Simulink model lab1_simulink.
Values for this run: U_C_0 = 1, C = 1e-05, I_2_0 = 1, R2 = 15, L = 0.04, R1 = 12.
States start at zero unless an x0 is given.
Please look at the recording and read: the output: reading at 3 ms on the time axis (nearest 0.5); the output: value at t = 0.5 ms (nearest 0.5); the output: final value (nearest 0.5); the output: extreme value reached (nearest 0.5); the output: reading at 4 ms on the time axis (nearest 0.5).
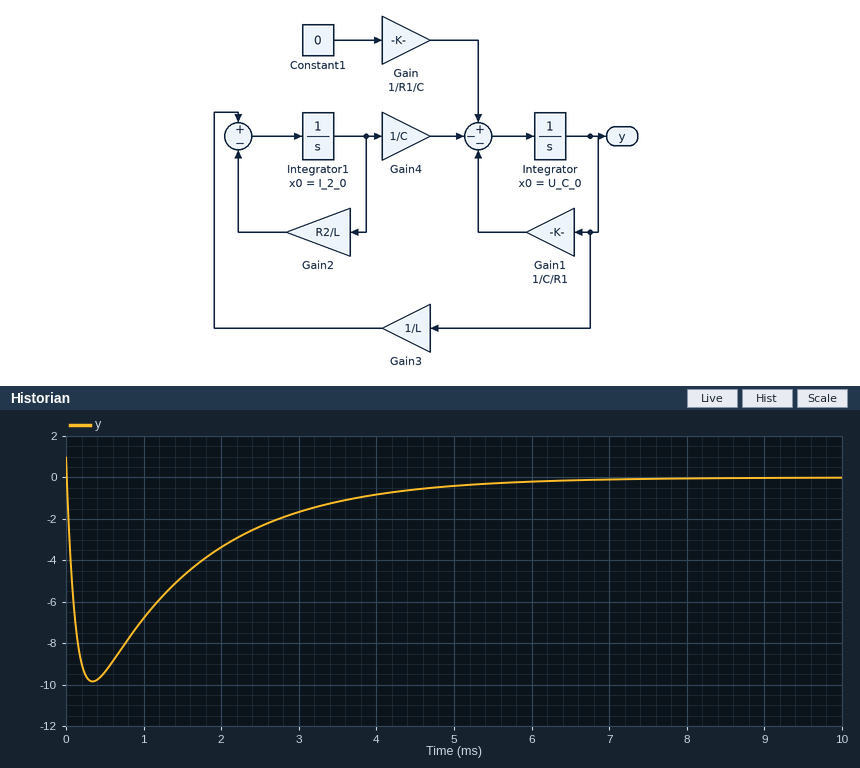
-1.5
-9.5
0.0
-10.0
-1.0
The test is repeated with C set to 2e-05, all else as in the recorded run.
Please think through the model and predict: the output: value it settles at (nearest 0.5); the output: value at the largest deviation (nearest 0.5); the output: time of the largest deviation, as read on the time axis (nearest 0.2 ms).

0.0
-9.0
0.6 ms
